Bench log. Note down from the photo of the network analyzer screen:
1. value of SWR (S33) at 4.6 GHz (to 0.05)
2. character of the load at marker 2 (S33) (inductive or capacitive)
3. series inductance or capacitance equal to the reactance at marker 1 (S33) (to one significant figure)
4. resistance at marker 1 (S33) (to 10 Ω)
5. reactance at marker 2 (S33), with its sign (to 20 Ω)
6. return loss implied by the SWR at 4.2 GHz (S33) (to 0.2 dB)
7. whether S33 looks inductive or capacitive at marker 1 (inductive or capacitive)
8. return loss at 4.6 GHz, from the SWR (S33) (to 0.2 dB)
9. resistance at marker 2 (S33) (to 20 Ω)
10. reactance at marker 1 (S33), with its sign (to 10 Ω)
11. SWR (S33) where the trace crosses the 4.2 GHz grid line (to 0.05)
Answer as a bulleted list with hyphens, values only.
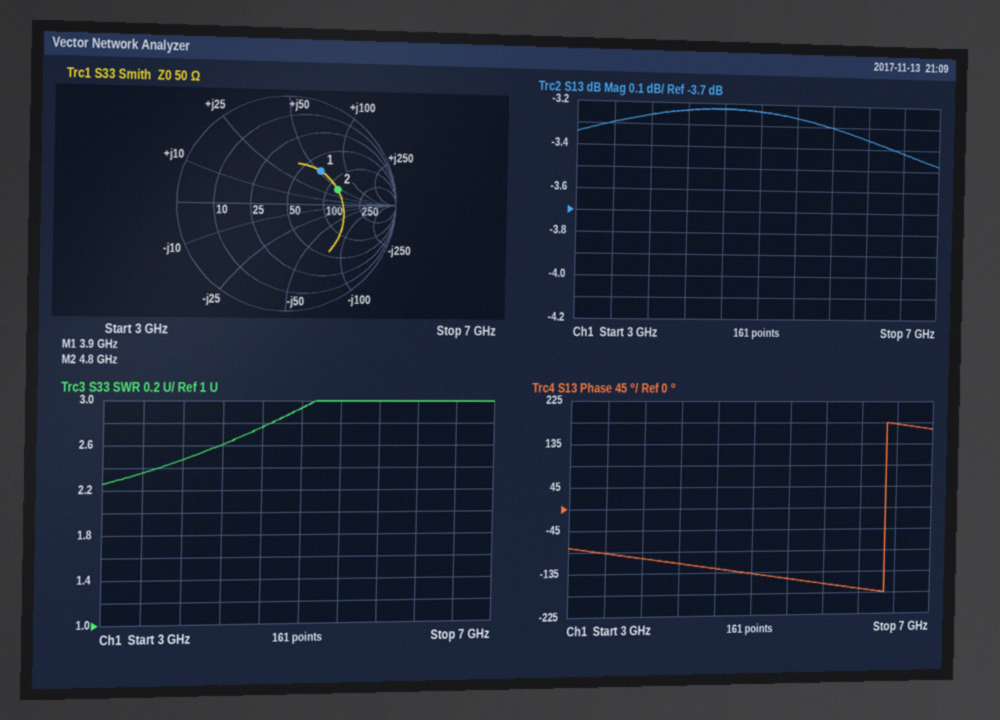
- 2.75
- inductive
- 2 nH
- 70 Ω
- +40 Ω
- 7.0 dB
- inductive
- 6.6 dB
- 120 Ω
- +50 Ω
- 2.60
